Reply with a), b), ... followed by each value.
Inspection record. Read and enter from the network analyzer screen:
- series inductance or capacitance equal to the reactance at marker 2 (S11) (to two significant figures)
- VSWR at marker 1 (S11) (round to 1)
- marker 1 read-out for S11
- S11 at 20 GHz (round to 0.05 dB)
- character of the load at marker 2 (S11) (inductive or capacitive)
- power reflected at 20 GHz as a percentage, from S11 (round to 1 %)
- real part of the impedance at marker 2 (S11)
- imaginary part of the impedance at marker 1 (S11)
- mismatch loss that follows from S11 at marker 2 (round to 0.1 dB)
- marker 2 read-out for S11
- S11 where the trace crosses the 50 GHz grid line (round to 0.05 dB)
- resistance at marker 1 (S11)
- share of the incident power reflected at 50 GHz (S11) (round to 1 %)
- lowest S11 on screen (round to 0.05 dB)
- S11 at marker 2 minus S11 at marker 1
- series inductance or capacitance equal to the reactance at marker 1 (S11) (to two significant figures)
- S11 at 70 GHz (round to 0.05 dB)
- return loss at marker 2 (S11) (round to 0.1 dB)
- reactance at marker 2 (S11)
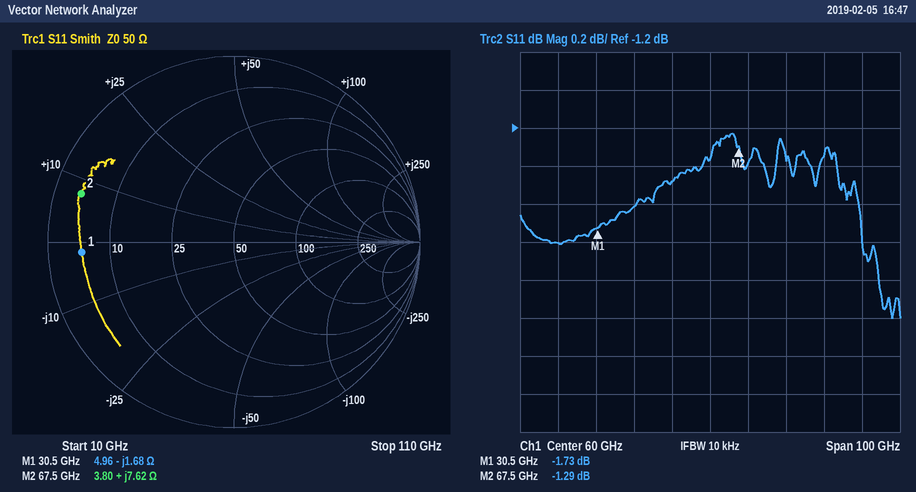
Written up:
a) 18 pH
b) 10
c) -1.73 dB
d) -1.80 dB
e) inductive
f) 66 %
g) 3.80 Ω
h) -1.68 Ω
i) 5.9 dB
j) -1.29 dB
k) -1.50 dB
l) 4.96 Ω
m) 71 %
n) -2.20 dB
o) 0.44 dB
p) 3.1 pF
q) -1.40 dB
r) 1.3 dB
s) +7.62 Ω
